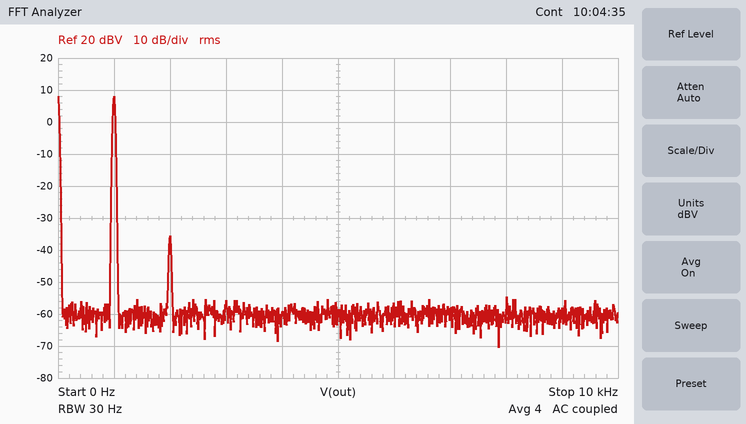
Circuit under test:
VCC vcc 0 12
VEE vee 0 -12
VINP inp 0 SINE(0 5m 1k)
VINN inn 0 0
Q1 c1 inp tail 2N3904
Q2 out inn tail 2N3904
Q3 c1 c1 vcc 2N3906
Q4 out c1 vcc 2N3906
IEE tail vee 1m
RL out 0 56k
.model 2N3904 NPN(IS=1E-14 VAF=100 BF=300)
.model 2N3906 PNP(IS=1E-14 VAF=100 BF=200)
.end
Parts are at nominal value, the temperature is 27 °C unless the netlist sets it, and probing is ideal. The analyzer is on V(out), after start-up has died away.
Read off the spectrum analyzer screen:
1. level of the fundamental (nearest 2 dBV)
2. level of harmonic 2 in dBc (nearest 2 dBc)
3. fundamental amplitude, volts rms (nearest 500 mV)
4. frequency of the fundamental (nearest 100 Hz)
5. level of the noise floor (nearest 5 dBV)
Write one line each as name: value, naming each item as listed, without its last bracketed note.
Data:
level of the fundamental: 8 dBV
level of harmonic 2 in dBc: -44 dBc
fundamental amplitude, volts rms: 2.5 V
frequency of the fundamental: 1.0 kHz
level of the noise floor: -60 dBV
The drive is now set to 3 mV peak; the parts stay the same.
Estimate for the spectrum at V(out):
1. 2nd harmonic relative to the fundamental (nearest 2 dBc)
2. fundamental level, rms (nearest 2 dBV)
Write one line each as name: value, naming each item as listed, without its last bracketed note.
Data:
2nd harmonic relative to the fundamental: -48 dBc
fundamental level, rms: 4 dBV
